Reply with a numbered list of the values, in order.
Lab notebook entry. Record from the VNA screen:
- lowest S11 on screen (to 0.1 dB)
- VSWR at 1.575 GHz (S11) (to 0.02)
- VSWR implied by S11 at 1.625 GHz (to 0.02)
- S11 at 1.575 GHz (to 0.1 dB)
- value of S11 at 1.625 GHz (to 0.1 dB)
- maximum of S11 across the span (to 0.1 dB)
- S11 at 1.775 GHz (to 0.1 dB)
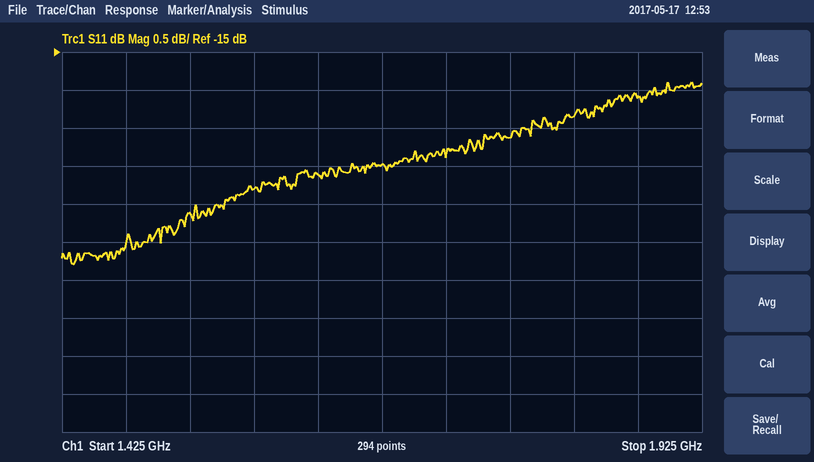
1. -17.8 dB
2. 1.34
3. 1.34
4. -16.8 dB
5. -16.6 dB
6. -15.4 dB
7. -16.1 dB
